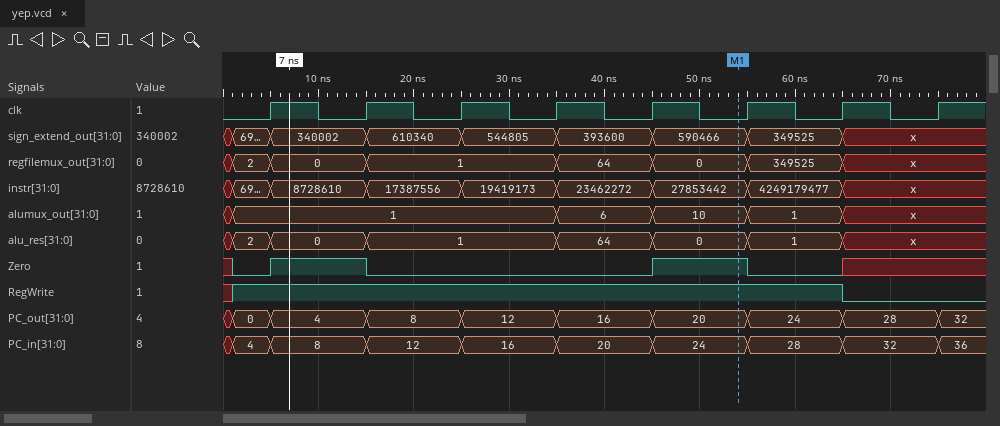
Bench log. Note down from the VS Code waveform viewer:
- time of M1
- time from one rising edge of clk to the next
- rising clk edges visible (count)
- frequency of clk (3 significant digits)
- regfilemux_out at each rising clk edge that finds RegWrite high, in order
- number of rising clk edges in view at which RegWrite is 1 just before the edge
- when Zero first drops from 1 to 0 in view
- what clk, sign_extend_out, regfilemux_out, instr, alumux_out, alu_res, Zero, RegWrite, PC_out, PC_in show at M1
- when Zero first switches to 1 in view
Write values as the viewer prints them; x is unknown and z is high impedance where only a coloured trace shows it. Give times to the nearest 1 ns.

54 ns
10 ns
8
100 MHz
2, 0, 1, 1, 64, 0, 349525
7
15 ns
clk=0, sign_extend_out=590466, regfilemux_out=0, instr=27853442, alumux_out=10, alu_res=0, Zero=1, RegWrite=1, PC_out=20, PC_in=24
5 ns
